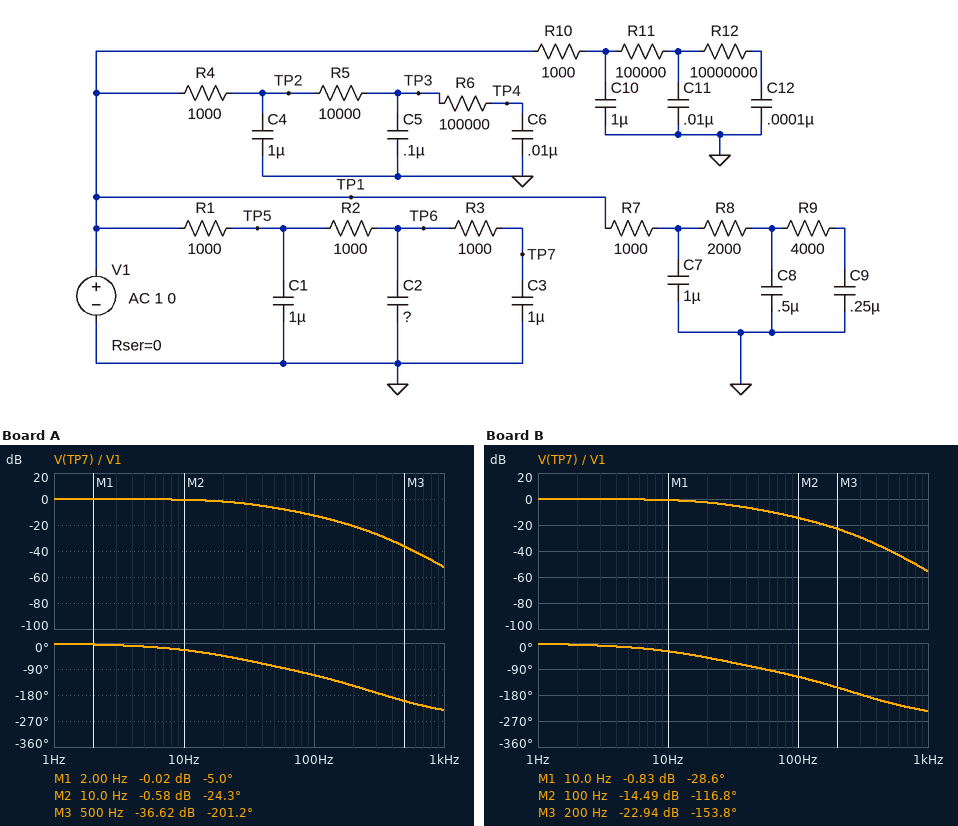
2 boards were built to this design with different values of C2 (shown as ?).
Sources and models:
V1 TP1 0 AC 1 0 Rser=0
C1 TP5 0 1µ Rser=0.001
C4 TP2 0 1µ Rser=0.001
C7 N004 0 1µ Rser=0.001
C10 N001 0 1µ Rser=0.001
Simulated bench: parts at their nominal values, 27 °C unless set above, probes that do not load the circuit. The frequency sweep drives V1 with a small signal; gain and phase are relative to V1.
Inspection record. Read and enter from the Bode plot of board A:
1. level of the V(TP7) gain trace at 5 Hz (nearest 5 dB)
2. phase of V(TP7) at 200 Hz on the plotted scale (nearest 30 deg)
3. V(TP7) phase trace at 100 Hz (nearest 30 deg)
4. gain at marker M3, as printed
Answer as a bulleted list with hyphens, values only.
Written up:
- 0 dB
- -150 deg
- -120 deg
- -36.62 dB
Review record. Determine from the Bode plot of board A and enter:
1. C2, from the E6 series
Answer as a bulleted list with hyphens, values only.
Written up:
- 1.5 µF
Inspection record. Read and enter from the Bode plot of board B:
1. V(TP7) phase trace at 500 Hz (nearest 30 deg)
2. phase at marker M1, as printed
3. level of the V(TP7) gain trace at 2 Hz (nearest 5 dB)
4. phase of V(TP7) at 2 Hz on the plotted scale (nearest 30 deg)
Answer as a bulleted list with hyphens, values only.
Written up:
- -210 deg
- -28.6 deg
- 0 dB
- 0 deg
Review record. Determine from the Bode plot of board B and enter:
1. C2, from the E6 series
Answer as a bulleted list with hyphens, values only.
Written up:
- 2.2 µF
